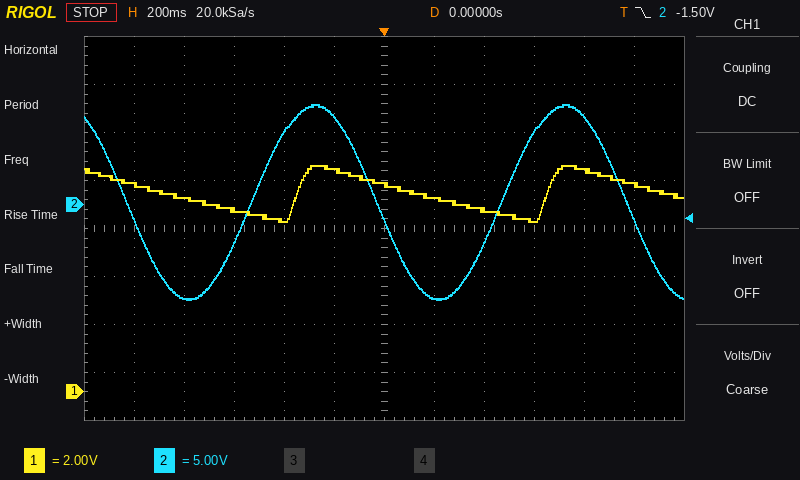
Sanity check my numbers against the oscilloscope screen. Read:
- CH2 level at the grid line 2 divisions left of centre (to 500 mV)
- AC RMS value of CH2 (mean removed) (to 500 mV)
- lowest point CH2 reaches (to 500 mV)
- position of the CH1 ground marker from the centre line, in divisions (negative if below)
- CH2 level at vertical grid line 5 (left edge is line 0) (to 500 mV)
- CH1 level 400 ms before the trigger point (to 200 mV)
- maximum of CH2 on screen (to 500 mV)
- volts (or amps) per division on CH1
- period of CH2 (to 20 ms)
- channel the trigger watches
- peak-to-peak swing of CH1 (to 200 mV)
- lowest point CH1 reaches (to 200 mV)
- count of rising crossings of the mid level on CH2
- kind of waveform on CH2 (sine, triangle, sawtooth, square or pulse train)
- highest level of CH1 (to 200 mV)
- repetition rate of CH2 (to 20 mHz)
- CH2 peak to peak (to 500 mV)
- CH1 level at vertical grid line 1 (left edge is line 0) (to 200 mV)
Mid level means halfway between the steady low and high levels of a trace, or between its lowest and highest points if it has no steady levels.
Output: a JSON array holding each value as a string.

["7.5 V", "7.0 V", "-10.0 V", "-3.4 div", "9.0 V", "7.2 V", "10.5 V", "2 V", "1.00 s", "CH2", "2.4 V", "7.0 V", "2", "sine", "9.4 V", "1.00 Hz", "20.5 V", "8.6 V"]
